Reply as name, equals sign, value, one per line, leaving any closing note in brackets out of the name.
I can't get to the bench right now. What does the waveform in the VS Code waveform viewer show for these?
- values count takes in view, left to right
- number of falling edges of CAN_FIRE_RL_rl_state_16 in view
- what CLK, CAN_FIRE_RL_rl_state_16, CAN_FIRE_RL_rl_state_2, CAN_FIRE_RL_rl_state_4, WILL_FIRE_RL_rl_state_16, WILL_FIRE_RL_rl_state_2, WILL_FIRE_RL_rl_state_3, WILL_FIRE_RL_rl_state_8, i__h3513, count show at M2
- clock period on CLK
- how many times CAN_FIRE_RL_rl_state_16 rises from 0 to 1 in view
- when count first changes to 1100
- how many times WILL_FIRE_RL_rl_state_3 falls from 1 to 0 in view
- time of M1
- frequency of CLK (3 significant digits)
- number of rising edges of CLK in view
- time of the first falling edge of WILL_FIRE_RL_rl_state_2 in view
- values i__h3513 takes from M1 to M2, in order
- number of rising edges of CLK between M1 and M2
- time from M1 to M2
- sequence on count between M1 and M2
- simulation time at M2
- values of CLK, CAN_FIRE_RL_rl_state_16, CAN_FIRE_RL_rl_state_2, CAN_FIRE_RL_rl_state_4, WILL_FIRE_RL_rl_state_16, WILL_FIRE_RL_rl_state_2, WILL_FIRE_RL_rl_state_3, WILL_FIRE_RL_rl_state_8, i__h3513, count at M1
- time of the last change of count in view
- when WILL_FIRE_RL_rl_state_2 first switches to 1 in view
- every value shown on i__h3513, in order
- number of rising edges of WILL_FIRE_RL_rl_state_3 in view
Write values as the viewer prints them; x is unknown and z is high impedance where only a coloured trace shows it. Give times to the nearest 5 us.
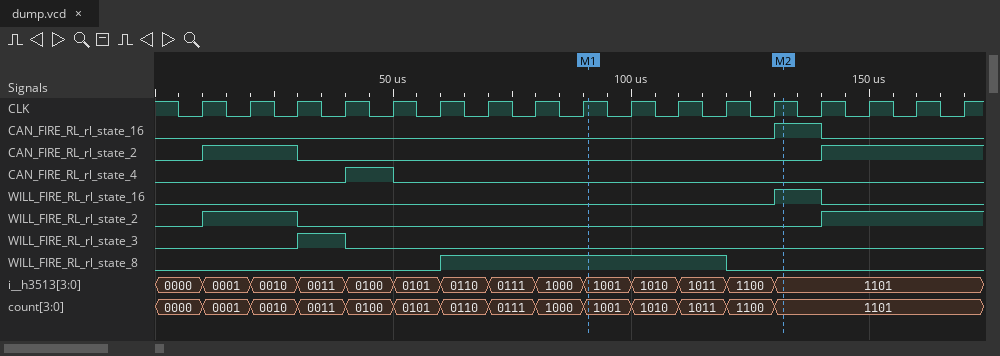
values count takes in view, left to right = 0000, 0001, 0010, 0011, 0100, 0101, 0110, 0111, 1000, 1001, 1010, 1011, 1100, 1101
number of falling edges of CAN_FIRE_RL_rl_state_16 in view = 1
what CLK, CAN_FIRE_RL_rl_state_16, CAN_FIRE_RL_rl_state_2, CAN_FIRE_RL_rl_state_4, WILL_FIRE_RL_rl_state_16, WILL_FIRE_RL_rl_state_2, WILL_FIRE_RL_rl_state_3, WILL_FIRE_RL_rl_state_8, i__h3513, count show at M2 = CLK=1, CAN_FIRE_RL_rl_state_16=1, CAN_FIRE_RL_rl_state_2=0, CAN_FIRE_RL_rl_state_4=0, WILL_FIRE_RL_rl_state_16=1, WILL_FIRE_RL_rl_state_2=0, WILL_FIRE_RL_rl_state_3=0, WILL_FIRE_RL_rl_state_8=0, i__h3513=1101, count=1101
clock period on CLK = 10 us
how many times CAN_FIRE_RL_rl_state_16 rises from 0 to 1 in view = 1
when count first changes to 1100 = 120 us
how many times WILL_FIRE_RL_rl_state_3 falls from 1 to 0 in view = 1
time of M1 = 90 us
frequency of CLK = 100 kHz
number of rising edges of CLK in view = 17
time of the first falling edge of WILL_FIRE_RL_rl_state_2 in view = 30 us
values i__h3513 takes from M1 to M2, in order = 1001, 1010, 1011, 1100, 1101
number of rising edges of CLK between M1 and M2 = 4
time from M1 to M2 = 40 us
sequence on count between M1 and M2 = 1001, 1010, 1011, 1100, 1101
simulation time at M2 = 130 us
values of CLK, CAN_FIRE_RL_rl_state_16, CAN_FIRE_RL_rl_state_2, CAN_FIRE_RL_rl_state_4, WILL_FIRE_RL_rl_state_16, WILL_FIRE_RL_rl_state_2, WILL_FIRE_RL_rl_state_3, WILL_FIRE_RL_rl_state_8, i__h3513, count at M1 = CLK=1, CAN_FIRE_RL_rl_state_16=0, CAN_FIRE_RL_rl_state_2=0, CAN_FIRE_RL_rl_state_4=0, WILL_FIRE_RL_rl_state_16=0, WILL_FIRE_RL_rl_state_2=0, WILL_FIRE_RL_rl_state_3=0, WILL_FIRE_RL_rl_state_8=1, i__h3513=1001, count=1001
time of the last change of count in view = 130 us
when WILL_FIRE_RL_rl_state_2 first switches to 1 in view = 10 us
every value shown on i__h3513, in order = 0000, 0001, 0010, 0011, 0100, 0101, 0110, 0111, 1000, 1001, 1010, 1011, 1100, 1101
number of rising edges of WILL_FIRE_RL_rl_state_3 in view = 1
